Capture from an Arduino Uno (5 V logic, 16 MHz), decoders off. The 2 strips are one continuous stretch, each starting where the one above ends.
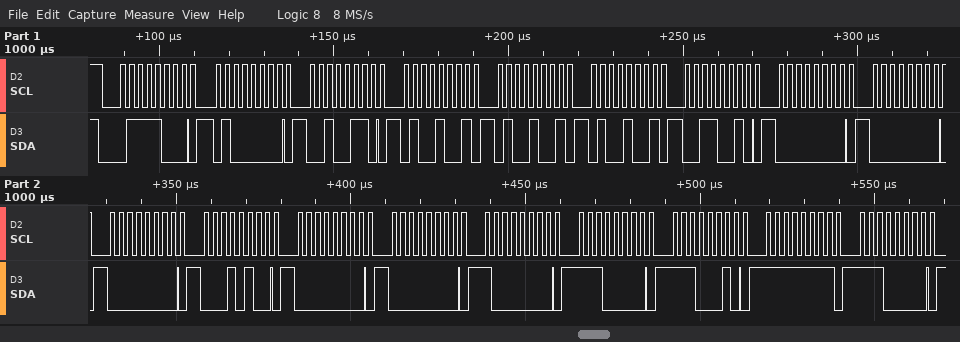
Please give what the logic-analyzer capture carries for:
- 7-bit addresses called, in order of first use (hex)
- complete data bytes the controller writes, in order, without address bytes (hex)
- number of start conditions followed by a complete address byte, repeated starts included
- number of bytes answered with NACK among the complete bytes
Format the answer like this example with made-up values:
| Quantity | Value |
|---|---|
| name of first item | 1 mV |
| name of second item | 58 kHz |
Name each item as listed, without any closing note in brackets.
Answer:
| Quantity | Value |
|---|---|
| 7-bit addresses called, in order of first use | 0x3C |
| complete data bytes the controller writes, in order, without address bytes | 40 26 49 49 49 32 00 00 00 14 00 00 80 E0 E2 FF E0 |
| number of start conditions followed by a complete address byte, repeated starts included | 1 |
| number of bytes answered with NACK among the complete bytes | 0 |
